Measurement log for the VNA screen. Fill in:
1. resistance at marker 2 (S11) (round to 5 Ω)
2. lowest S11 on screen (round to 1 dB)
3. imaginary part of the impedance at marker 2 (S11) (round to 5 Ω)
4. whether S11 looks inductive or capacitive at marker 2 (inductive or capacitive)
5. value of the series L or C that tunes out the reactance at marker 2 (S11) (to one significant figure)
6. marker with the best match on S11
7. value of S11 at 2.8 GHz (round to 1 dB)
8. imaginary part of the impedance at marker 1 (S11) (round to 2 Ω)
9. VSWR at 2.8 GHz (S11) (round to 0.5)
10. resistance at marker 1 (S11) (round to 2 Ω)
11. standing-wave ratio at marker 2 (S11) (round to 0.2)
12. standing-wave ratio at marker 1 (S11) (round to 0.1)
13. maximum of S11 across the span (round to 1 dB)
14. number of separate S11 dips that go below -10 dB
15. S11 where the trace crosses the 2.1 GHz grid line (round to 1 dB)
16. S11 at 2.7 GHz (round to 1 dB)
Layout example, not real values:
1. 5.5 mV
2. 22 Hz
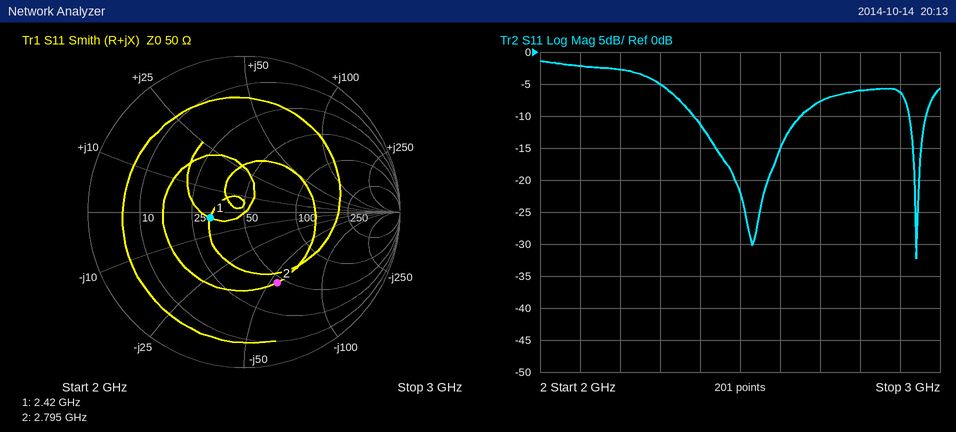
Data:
1. 45 Ω
2. -32 dB
3. -55 Ω
4. capacitive
5. 3 nH
6. marker 1
7. -6 dB
8. -2 Ω
9. 3.0
10. 32 Ω
11. 3.0
12. 1.6
13. -1 dB
14. 2
15. -2 dB
16. -8 dB
